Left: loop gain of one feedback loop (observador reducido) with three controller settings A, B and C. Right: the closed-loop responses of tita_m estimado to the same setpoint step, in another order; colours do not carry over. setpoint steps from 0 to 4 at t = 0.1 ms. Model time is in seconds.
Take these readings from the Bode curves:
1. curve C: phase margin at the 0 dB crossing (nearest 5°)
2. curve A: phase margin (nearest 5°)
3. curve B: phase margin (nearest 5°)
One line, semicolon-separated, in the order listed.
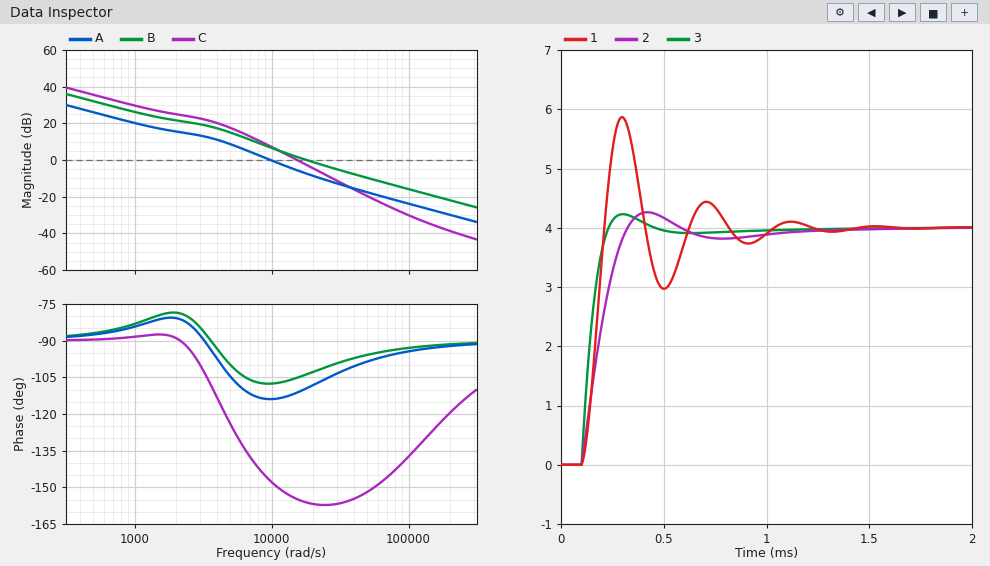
25°; 65°; 75°
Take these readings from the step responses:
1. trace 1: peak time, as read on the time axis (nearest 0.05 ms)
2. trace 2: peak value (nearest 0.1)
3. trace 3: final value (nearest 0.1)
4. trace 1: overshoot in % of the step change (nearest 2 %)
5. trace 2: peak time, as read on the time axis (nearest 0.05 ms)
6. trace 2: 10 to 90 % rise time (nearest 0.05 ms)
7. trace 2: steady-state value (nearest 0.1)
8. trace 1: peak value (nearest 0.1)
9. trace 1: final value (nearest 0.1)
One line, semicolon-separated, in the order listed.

0.30 ms; 4.3; 4.0; 46 %; 0.40 ms; 0.15 ms; 4.0; 5.9; 4.0
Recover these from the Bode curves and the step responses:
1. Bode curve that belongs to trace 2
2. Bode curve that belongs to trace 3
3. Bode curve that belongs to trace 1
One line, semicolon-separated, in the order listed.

A; B; C
